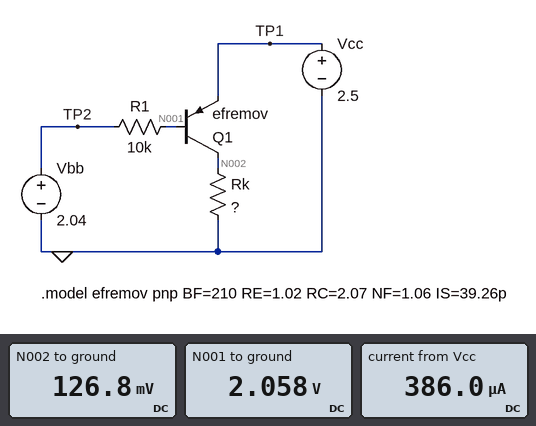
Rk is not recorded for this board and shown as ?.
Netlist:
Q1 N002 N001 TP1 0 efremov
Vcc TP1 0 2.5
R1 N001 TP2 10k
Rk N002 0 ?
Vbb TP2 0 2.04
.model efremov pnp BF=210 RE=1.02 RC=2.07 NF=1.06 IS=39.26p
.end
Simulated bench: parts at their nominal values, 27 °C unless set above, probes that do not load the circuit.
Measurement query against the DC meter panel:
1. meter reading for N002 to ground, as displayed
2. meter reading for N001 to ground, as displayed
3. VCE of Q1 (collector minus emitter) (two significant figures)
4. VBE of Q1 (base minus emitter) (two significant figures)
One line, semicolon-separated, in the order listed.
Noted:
126.8 mV; 2.058 V; -2.4 V; -440 mV
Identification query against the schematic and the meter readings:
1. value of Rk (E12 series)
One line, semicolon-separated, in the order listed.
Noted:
330 Ω
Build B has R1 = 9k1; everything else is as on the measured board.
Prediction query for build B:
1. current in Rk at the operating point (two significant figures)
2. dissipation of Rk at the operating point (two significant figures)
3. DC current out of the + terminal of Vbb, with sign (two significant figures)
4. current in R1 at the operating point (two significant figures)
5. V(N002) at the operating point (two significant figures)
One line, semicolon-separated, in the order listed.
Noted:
400 µA; 52 µW; -1.9 µA; 1.9 µA; 130 mV
